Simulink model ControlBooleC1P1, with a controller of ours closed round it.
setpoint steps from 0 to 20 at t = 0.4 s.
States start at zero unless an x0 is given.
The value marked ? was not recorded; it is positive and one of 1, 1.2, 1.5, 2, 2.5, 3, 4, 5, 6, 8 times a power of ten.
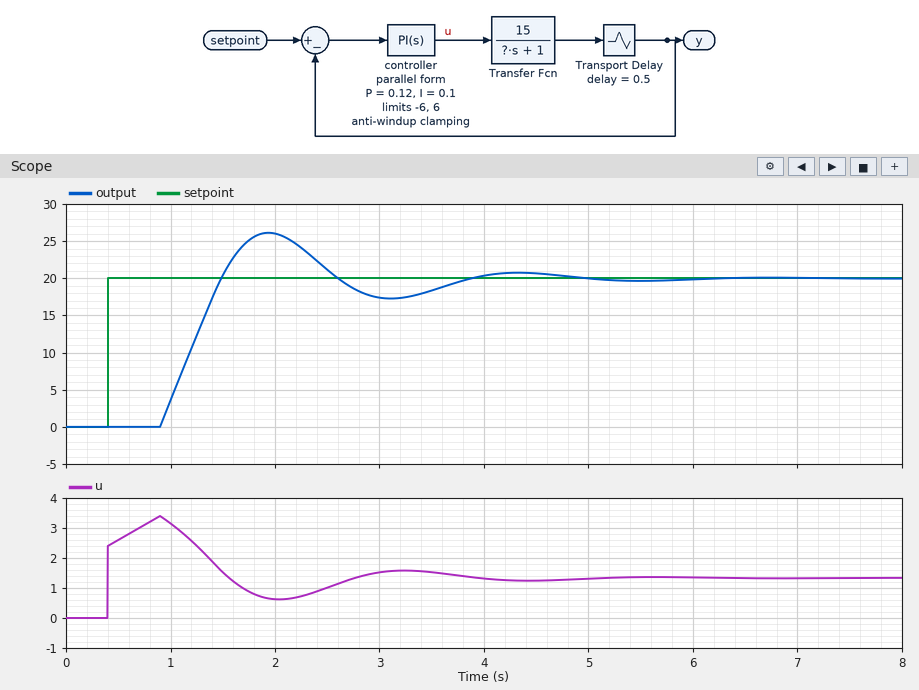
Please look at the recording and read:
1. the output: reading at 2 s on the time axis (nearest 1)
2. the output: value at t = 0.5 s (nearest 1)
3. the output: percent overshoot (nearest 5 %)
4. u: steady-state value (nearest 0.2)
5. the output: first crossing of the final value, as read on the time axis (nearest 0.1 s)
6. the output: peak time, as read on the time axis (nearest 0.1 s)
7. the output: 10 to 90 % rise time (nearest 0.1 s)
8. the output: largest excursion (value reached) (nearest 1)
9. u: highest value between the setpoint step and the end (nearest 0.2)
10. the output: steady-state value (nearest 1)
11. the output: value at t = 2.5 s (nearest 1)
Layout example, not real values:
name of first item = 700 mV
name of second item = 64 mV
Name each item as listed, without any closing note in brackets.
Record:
the output: reading at 2 s on the time axis = 26
the output: value at t = 0.5 s = 0
the output: percent overshoot = 30 %
u: steady-state value = 1.4
the output: first crossing of the final value, as read on the time axis = 1.5 s
the output: peak time, as read on the time axis = 1.9 s
the output: 10 to 90 % rise time = 0.5 s
the output: largest excursion (value reached) = 26
u: highest value between the setpoint step and the end = 3.4
the output: steady-state value = 20
the output: value at t = 2.5 s = 21
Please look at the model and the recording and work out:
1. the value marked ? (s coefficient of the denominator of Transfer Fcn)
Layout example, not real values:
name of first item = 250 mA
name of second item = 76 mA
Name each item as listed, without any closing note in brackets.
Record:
the value marked ? = 1
